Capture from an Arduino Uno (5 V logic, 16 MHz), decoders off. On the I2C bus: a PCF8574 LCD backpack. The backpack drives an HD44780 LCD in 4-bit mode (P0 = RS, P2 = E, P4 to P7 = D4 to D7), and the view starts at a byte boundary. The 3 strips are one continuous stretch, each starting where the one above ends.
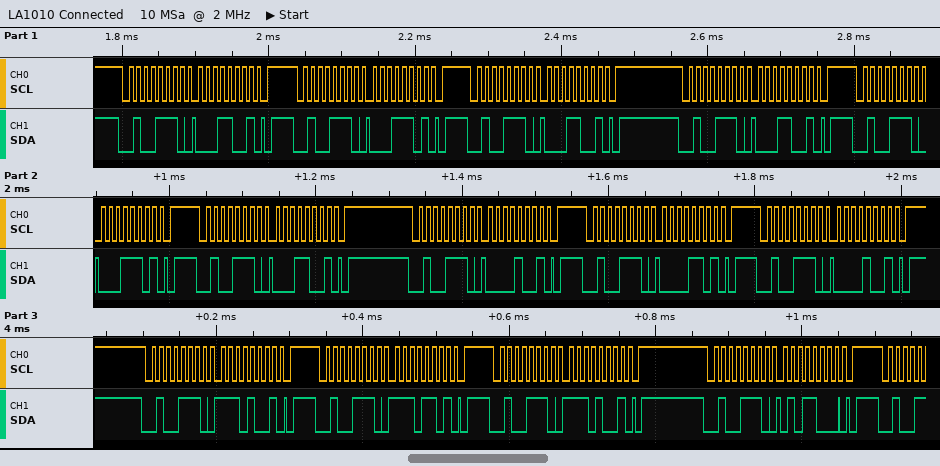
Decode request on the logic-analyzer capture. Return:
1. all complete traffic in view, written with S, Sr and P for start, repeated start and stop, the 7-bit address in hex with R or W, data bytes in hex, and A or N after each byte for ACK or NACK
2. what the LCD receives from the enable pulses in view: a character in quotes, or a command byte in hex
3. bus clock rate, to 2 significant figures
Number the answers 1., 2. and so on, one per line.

1. S 27W A 19 A P S 27W A 1D A P S 27W A 19 A P S 27W A 19 A P S 27W A 1D A P S 27W A 19 A P S 27W A 09 A P S 27W A 0D A P S 27W A 09 A P S 27W A E9 A P S 27W A ED A P S 27W A E9 A P S 27W A 58 A P
2. data 0x11 data 0x0E
3. 100 kHz
